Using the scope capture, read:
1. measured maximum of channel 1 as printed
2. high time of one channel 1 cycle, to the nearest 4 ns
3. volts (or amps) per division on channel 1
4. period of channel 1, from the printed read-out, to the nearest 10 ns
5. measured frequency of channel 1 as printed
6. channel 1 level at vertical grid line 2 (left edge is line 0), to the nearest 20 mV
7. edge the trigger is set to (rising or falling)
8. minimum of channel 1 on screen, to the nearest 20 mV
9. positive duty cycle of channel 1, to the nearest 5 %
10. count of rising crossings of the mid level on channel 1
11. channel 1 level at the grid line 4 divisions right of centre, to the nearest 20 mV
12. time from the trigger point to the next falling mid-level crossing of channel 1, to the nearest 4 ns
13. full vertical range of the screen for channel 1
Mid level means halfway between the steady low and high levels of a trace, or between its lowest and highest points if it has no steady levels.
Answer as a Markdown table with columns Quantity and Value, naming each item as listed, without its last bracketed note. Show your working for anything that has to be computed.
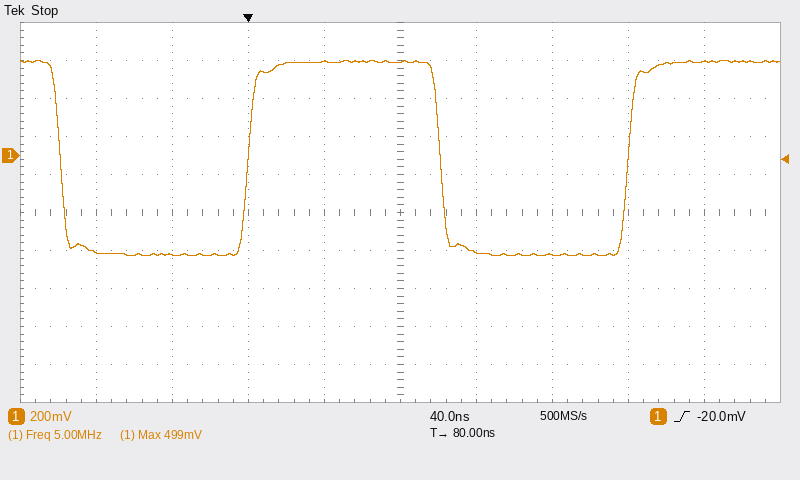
| Quantity | Value |
|---|---|
| measured maximum of channel 1 as printed | 499 mV |
| high time of one channel 1 cycle, to the nearest 4 ns | 100 ns |
| volts (or amps) per division on channel 1 | 200 mV |
| period of channel 1, from the printed read-out, to the nearest 10 ns | 1 / 5.00 MHz ≈ 200 ns |
| measured frequency of channel 1 as printed | 5.00 MHz |
| channel 1 level at vertical grid line 2 (left edge is line 0), to the nearest 20 mV | -520 mV |
| edge the trigger is set to | rising |
| minimum of channel 1 on screen, to the nearest 20 mV | -520 mV |
| positive duty cycle of channel 1, to the nearest 5 % | 50 % |
| count of rising crossings of the mid level on channel 1 | 2 |
| channel 1 level at the grid line 4 divisions right of centre, to the nearest 20 mV | 500 mV |
| time from the trigger point to the next falling mid-level crossing of channel 1, to the nearest 4 ns | 100 ns |
| full vertical range of the screen for channel 1 | 2 V |
